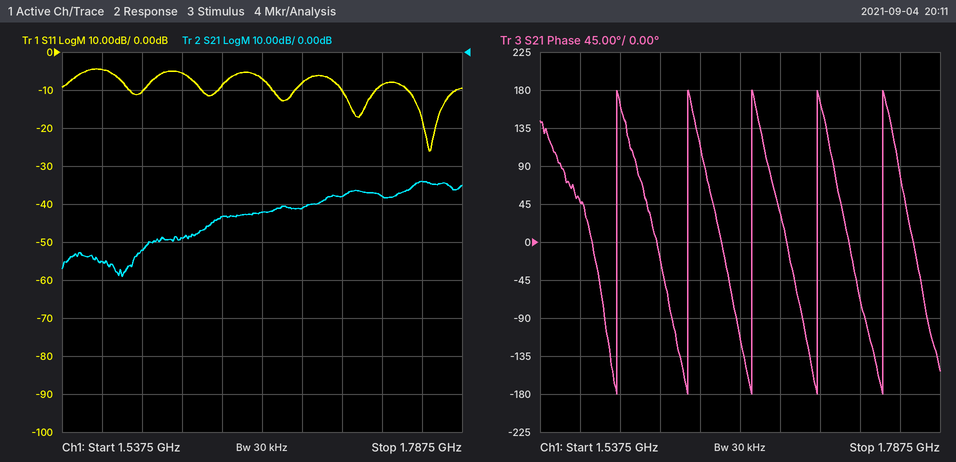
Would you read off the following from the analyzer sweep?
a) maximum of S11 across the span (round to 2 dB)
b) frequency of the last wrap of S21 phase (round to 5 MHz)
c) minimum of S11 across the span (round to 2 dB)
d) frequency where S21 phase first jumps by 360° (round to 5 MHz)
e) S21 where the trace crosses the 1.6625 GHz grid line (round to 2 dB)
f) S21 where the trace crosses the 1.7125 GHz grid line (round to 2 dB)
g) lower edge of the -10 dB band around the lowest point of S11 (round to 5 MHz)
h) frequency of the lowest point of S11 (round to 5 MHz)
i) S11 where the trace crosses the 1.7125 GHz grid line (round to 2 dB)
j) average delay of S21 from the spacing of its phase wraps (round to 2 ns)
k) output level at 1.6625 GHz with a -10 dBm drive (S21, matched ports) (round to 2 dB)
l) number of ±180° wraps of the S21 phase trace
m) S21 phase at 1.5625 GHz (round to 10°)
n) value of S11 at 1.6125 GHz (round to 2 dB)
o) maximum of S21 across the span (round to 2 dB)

-4 dB
1.750 GHz
-26 dB
1.585 GHz
-42 dB
-38 dB
1.755 GHz
1.765 GHz
-10 dB
24 ns
-52 dBm
5
50°
-6 dB
-34 dB
